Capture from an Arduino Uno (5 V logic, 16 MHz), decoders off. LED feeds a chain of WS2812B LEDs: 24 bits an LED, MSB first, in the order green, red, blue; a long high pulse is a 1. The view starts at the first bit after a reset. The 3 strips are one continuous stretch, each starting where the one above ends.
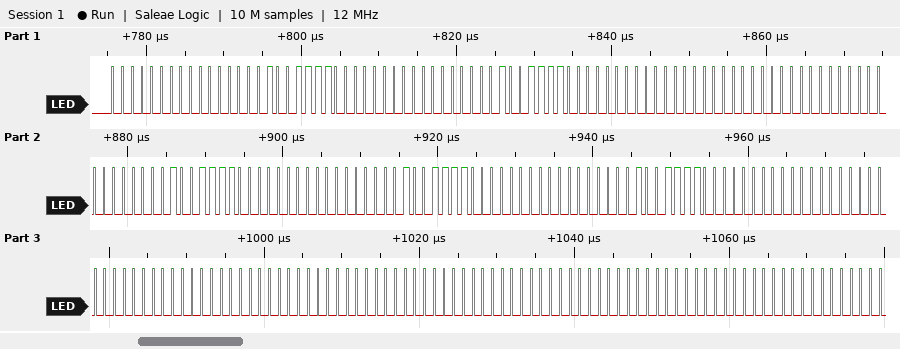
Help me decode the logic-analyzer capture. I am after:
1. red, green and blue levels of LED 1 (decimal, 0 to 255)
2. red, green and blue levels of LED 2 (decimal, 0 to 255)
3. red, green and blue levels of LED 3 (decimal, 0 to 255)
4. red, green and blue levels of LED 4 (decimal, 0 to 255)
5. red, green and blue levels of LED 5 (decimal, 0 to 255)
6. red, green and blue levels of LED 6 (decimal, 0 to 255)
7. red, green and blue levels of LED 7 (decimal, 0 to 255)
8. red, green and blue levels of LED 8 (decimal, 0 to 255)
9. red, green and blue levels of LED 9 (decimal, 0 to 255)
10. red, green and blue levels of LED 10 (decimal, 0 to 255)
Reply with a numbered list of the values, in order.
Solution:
1. 0, 0, 158
2. 0, 0, 158
3. 0, 0, 0
4. 0, 0, 158
5. 0, 0, 158
6. 0, 0, 158
7. 0, 0, 0
8. 0, 0, 0
9. 0, 0, 0
10. 0, 0, 0
